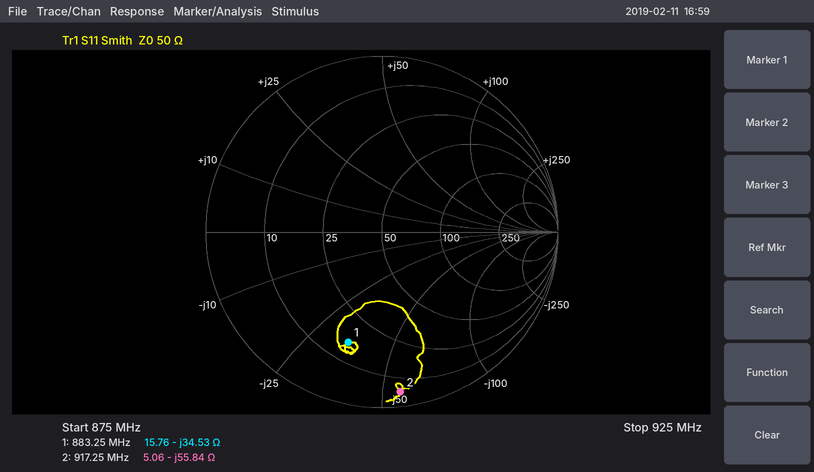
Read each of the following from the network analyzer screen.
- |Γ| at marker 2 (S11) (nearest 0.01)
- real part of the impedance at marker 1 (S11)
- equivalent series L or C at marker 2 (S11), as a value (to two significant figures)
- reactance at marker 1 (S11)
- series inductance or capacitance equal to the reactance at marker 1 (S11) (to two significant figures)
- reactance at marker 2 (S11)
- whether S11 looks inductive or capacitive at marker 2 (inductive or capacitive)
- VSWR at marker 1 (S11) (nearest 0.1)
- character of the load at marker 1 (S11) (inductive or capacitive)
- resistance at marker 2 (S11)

0.91
15.76 Ω
3.1 pF
-34.53 Ω
5.2 pF
-55.84 Ω
capacitive
4.8
capacitive
5.06 Ω
